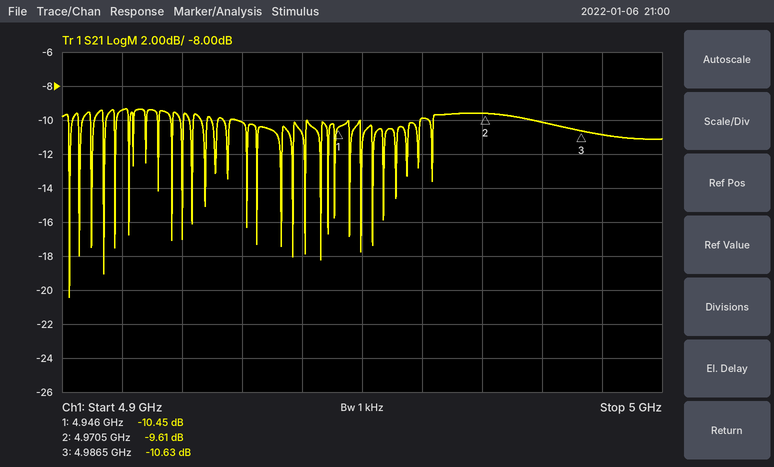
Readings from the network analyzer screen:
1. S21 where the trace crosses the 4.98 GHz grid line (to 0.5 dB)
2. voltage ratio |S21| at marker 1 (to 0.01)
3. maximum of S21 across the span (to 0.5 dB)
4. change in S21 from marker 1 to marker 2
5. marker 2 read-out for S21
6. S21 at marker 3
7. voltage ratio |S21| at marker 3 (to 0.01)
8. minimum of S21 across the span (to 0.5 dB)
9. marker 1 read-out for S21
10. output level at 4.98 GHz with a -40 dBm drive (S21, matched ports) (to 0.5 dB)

-10.0 dB
0.30
-9.5 dB
0.84 dB
-9.61 dB
-10.63 dB
0.29
-20.5 dB
-10.45 dB
-50.0 dBm
